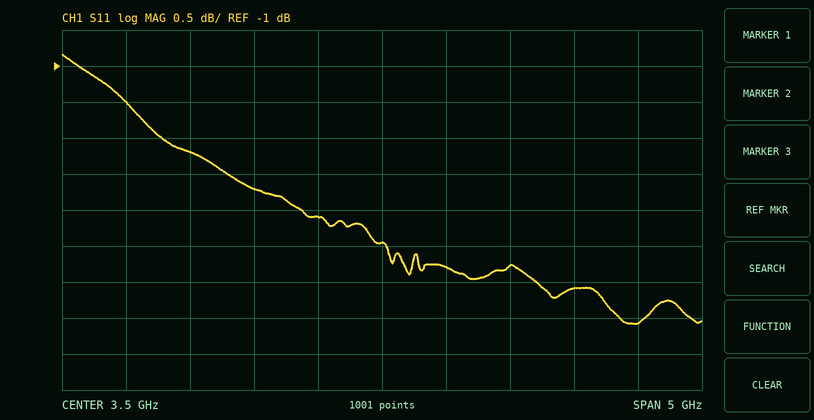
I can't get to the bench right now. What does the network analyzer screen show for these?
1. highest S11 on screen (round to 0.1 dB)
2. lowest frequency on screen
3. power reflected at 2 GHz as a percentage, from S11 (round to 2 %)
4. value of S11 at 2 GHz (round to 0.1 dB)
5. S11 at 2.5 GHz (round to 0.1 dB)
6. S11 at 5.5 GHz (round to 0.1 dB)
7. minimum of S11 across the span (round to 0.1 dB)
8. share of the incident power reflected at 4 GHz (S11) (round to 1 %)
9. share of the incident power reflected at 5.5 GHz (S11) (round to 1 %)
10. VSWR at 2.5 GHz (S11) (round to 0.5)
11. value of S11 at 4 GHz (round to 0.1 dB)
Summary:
-0.8 dB
1 GHz
60 %
-2.2 dB
-2.7 dB
-4.6 dB
-4.6 dB
42 %
35 %
6.5
-3.8 dB
